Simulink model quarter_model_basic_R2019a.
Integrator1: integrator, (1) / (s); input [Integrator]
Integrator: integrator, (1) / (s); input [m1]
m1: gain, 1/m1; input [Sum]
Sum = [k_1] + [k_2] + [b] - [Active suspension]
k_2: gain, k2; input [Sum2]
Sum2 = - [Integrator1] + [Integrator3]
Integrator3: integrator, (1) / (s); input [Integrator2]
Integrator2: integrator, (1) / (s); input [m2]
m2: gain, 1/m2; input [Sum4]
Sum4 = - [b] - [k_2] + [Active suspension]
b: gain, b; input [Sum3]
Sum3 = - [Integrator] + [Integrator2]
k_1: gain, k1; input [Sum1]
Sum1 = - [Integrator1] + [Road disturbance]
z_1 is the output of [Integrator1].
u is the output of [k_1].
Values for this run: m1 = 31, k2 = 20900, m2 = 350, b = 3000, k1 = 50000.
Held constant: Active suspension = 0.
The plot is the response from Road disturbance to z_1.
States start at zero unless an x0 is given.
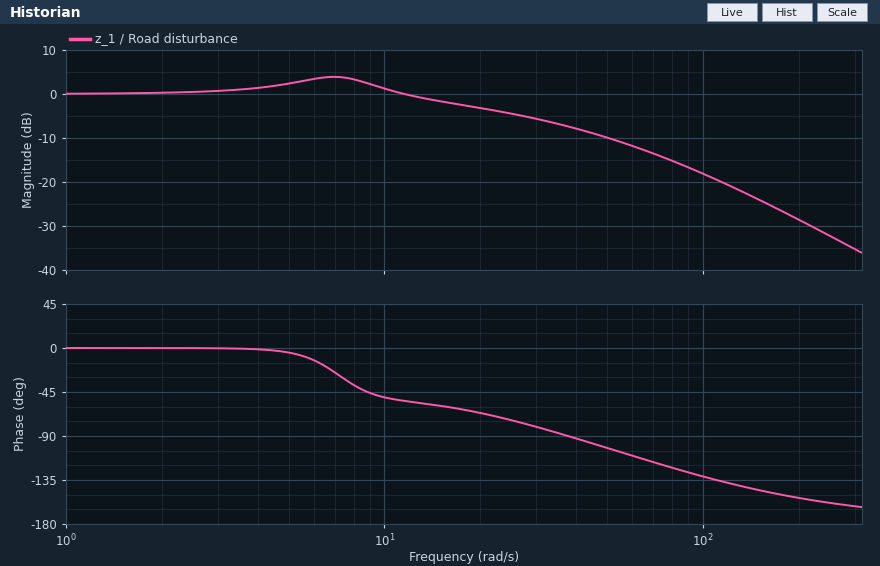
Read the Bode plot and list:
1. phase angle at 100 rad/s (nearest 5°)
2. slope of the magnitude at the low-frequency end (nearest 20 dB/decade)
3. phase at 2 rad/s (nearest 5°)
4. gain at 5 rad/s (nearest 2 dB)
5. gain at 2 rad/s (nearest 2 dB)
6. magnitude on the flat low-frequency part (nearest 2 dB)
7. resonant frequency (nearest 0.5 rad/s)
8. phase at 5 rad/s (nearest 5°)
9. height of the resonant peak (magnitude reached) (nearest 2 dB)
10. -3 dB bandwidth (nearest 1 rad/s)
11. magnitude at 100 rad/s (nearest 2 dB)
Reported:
-130°
0 dB/decade
0°
2 dB
0 dB
0 dB
7.0 rad/s
-5°
4 dB
19 rad/s
-18 dB
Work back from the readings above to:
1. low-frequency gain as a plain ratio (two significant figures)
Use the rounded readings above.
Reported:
1.0
